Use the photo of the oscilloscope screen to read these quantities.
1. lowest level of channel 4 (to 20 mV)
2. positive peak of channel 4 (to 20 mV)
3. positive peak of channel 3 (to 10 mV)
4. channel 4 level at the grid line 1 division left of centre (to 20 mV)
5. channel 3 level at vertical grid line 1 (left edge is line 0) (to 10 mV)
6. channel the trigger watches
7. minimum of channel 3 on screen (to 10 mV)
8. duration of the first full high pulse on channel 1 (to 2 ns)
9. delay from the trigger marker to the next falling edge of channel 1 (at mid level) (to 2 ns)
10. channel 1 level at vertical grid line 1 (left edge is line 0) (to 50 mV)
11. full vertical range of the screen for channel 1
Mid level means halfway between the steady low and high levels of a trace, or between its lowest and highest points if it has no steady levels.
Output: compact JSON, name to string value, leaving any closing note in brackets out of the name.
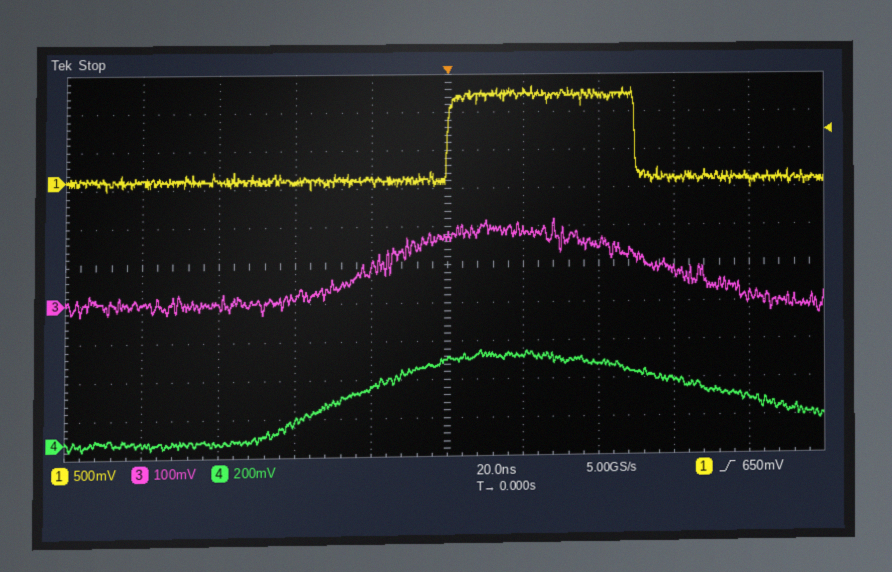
{"lowest level of channel 4": "-40 mV", "positive peak of channel 4": "480 mV", "positive peak of channel 3": "220 mV", "channel 4 level at the grid line 1 division left of centre": "280 mV", "channel 3 level at vertical grid line 1 (left edge is line 0)": "0 mV", "channel the trigger watches": "channel 1", "minimum of channel 3 on screen": "-30 mV", "duration of the first full high pulse on channel 1": "50 ns", "delay from the trigger marker to the next falling edge of channel 1 (at mid level)": "50 ns", "channel 1 level at vertical grid line 1 (left edge is line 0)": "0 mV", "full vertical range of the screen for channel 1": "5 V"}
